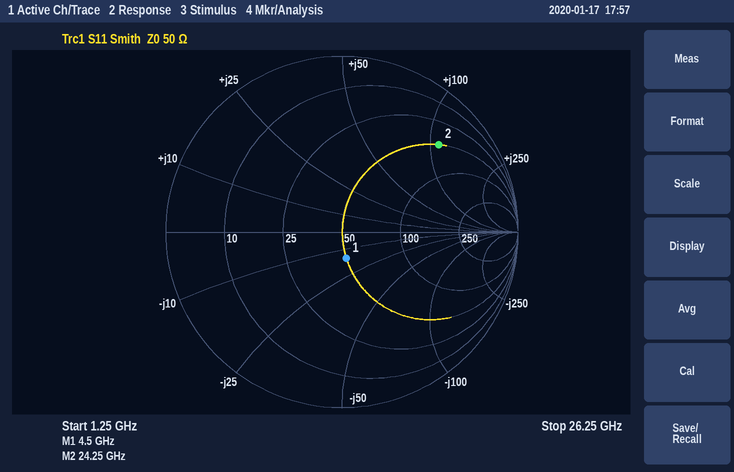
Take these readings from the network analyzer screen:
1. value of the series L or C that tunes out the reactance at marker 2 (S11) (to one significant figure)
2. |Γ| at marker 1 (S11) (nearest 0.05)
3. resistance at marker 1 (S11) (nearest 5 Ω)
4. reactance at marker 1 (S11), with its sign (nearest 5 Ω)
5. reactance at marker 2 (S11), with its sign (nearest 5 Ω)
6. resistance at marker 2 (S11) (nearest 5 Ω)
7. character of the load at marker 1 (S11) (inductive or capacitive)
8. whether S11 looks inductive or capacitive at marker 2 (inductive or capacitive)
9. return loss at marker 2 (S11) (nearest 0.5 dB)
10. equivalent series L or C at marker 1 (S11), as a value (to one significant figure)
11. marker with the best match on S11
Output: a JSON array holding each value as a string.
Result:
["60 fF", "0.15", "50 Ω", "-15 Ω", "+110 Ω", "50 Ω", "capacitive", "inductive", "2.5 dB", "2 pF", "marker 1"]
